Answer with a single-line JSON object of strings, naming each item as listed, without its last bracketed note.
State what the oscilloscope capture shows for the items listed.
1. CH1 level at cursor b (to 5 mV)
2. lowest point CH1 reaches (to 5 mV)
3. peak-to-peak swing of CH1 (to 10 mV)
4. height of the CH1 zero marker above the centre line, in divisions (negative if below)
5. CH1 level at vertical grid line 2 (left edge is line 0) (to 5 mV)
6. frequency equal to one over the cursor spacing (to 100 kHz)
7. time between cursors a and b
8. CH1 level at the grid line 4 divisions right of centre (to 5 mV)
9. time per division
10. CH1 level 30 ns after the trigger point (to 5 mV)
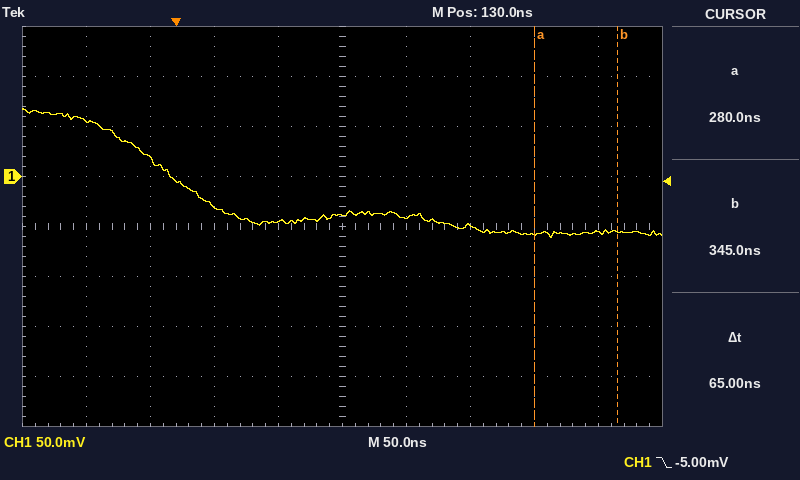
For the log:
{"CH1 level at cursor b": "-55 mV", "lowest point CH1 reaches": "-60 mV", "peak-to-peak swing of CH1": "130 mV", "height of the CH1 zero marker above the centre line, in divisions": "+1.0 div", "CH1 level at vertical grid line 2 (left edge is line 0)": "20 mV", "frequency equal to one over the cursor spacing": "15.4 MHz", "time between cursors a and b": "65 ns", "CH1 level at the grid line 4 divisions right of centre": "-55 mV", "time per division": "50 ns", "CH1 level 30 ns after the trigger point": "-30 mV"}
